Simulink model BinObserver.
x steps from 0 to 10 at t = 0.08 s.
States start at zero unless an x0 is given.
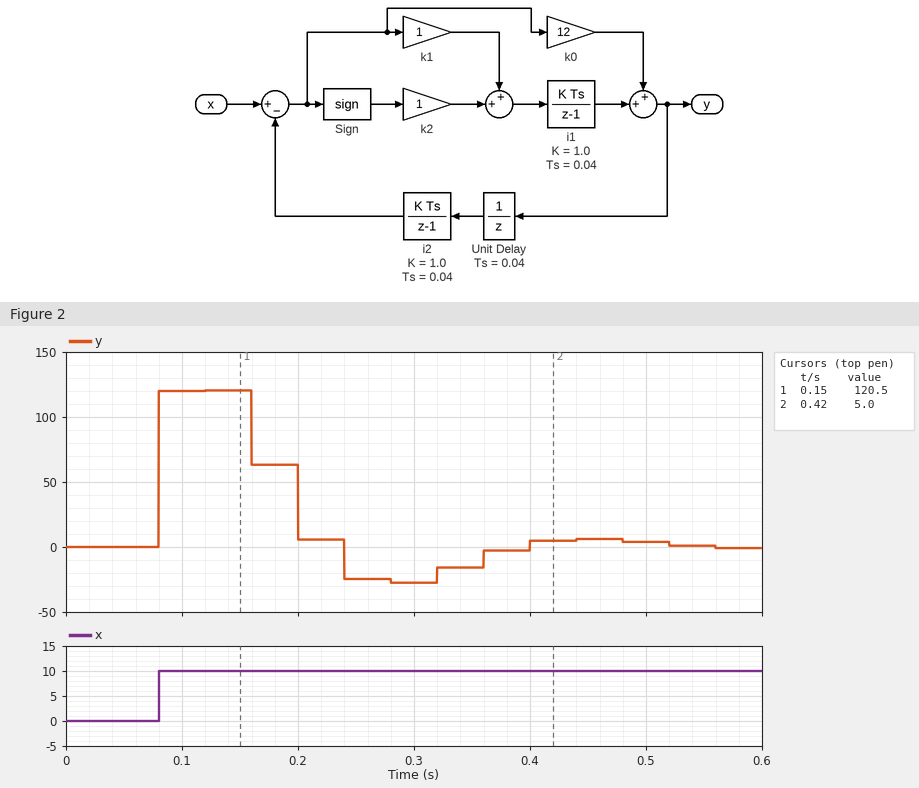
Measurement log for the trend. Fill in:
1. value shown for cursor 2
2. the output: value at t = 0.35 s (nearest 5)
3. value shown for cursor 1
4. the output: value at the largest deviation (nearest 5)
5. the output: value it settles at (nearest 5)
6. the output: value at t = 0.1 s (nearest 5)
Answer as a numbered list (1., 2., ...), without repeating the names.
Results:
1. 5.0
2. -15
3. 120.5
4. 120
5. 0
6. 120
